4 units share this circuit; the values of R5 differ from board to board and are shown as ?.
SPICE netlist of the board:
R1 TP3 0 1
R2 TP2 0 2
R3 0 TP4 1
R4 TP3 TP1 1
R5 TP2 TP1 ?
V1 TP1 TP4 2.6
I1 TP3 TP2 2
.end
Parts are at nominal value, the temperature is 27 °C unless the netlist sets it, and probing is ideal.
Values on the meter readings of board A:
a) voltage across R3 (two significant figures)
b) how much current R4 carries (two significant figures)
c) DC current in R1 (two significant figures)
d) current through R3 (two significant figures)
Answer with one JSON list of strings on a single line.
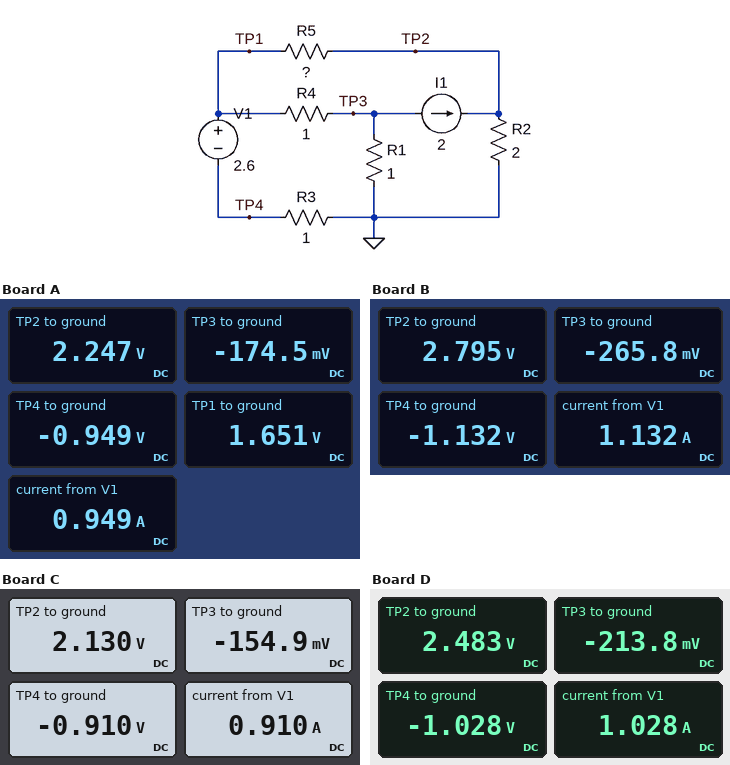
["950 mV", "1.8 A", "170 mA", "950 mA"]
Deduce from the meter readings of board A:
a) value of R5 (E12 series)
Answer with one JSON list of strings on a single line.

["0.68 Ω"]
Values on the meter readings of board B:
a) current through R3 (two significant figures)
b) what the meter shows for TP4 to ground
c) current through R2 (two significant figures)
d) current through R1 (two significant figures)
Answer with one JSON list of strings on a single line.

["1.1 A", "-1.132 V", "1.4 A", "270 mA"]
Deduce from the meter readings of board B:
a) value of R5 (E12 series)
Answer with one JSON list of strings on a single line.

["2.2 Ω"]
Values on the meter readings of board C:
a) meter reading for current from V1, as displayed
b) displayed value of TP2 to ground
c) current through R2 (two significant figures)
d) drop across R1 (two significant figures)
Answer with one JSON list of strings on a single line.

["0.910 A", "2.130 V", "1.1 A", "150 mV"]
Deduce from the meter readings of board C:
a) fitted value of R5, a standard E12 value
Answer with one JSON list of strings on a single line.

["0.47 Ω"]
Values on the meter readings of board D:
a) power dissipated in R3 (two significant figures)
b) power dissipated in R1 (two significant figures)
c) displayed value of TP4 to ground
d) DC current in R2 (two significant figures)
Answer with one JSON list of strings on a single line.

["1.1 W", "46 mW", "-1.028 V", "1.2 A"]
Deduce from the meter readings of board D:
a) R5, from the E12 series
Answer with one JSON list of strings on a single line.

["1.2 Ω"]
